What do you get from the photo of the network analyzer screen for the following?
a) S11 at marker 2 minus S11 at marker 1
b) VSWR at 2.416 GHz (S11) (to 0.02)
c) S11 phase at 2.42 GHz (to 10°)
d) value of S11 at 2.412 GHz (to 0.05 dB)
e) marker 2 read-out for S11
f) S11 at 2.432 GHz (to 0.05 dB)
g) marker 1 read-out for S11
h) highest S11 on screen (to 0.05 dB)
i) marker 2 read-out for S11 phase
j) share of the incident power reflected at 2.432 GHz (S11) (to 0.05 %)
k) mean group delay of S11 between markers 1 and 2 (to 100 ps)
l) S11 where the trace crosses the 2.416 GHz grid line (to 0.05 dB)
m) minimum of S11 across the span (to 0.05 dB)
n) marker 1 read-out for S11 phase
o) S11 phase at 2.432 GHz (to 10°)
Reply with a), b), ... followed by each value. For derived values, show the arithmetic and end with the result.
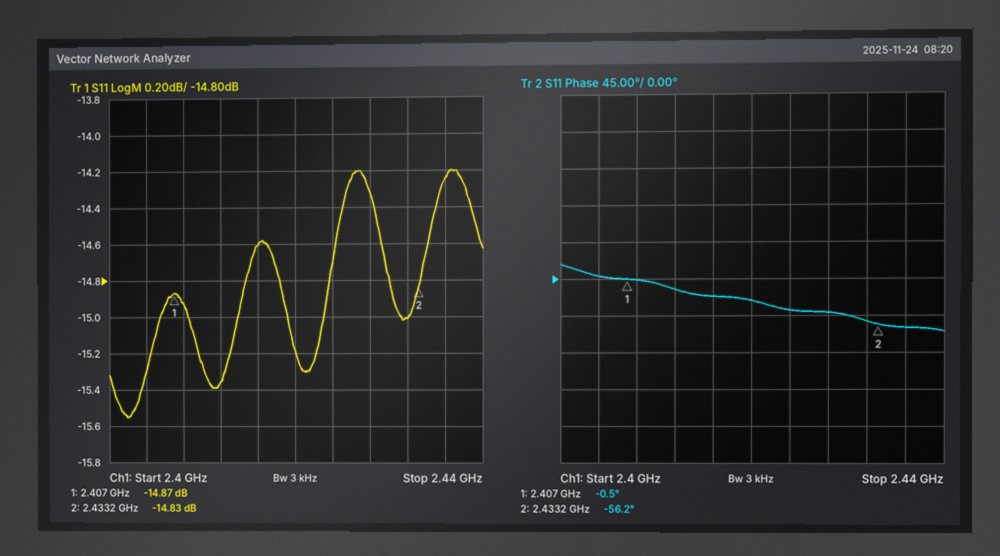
a) -14.83 − (-14.87) = 0.04 dB
b) |Γ| = 10^(-14.6/20) = 0.1862; VSWR = (1 + 0.1862)/(1 − 0.1862) ≈ 1.46
c) -30°
d) -15.35 dB
e) -14.83 dB
f) -15.00 dB
g) -14.87 dB
h) -14.20 dB
i) -56.2°
j) 10^(-15/10) ≈ 3.16 %, so 3.15 % to the nearest 0.05 %
k) −(-56.2° − (-0.5°))/(360° × 26.2 MHz) ≈ 5.9 ns
l) -14.60 dB
m) -15.55 dB
n) -0.5°
o) -50°
